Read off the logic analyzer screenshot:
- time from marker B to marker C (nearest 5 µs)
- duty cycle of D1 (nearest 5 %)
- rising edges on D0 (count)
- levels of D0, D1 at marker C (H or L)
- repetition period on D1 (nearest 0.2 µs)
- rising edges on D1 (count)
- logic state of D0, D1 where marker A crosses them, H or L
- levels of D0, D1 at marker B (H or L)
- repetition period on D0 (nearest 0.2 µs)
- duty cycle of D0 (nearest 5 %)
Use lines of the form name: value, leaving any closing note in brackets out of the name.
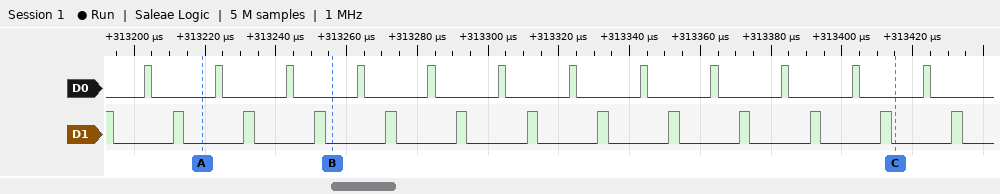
time from marker B to marker C: 160 µs
duty cycle of D1: 15 %
rising edges on D0: 12
levels of D0, D1 at marker C: D0=L, D1=L
repetition period on D1: 20 µs
rising edges on D1: 12
logic state of D0, D1 where marker A crosses them, H or L: D0=L, D1=L
levels of D0, D1 at marker B: D0=L, D1=L
repetition period on D0: 20 µs
duty cycle of D0: 10 %
